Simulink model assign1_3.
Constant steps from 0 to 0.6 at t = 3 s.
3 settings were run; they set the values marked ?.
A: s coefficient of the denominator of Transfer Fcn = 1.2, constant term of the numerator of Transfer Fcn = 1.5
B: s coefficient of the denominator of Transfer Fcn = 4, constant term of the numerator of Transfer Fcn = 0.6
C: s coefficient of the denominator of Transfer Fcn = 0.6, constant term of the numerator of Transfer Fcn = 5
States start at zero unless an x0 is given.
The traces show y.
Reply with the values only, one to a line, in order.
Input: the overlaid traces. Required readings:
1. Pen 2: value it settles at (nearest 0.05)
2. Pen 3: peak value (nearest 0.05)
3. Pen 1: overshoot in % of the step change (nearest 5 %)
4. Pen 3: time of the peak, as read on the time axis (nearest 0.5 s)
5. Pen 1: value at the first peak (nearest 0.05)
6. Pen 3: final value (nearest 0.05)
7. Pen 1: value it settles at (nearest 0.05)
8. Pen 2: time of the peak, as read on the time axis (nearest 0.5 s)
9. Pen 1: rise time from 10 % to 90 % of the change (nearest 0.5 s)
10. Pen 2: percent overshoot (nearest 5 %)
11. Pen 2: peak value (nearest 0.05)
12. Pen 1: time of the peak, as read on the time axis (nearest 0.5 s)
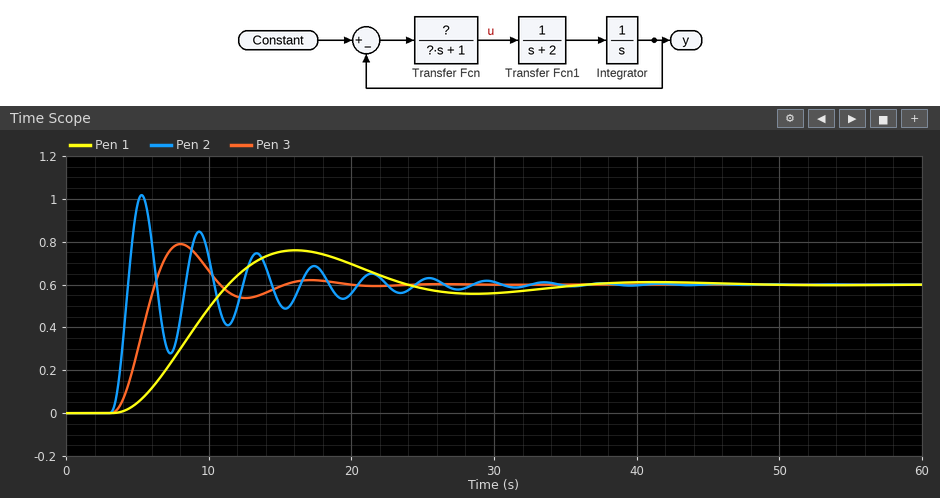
0.60
0.80
25 %
8.0 s
0.75
0.60
0.60
5.5 s
5.5 s
70 %
1.00
16.0 s
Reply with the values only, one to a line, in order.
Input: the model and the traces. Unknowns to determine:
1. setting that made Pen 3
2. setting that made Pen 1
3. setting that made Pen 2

A
B
C
